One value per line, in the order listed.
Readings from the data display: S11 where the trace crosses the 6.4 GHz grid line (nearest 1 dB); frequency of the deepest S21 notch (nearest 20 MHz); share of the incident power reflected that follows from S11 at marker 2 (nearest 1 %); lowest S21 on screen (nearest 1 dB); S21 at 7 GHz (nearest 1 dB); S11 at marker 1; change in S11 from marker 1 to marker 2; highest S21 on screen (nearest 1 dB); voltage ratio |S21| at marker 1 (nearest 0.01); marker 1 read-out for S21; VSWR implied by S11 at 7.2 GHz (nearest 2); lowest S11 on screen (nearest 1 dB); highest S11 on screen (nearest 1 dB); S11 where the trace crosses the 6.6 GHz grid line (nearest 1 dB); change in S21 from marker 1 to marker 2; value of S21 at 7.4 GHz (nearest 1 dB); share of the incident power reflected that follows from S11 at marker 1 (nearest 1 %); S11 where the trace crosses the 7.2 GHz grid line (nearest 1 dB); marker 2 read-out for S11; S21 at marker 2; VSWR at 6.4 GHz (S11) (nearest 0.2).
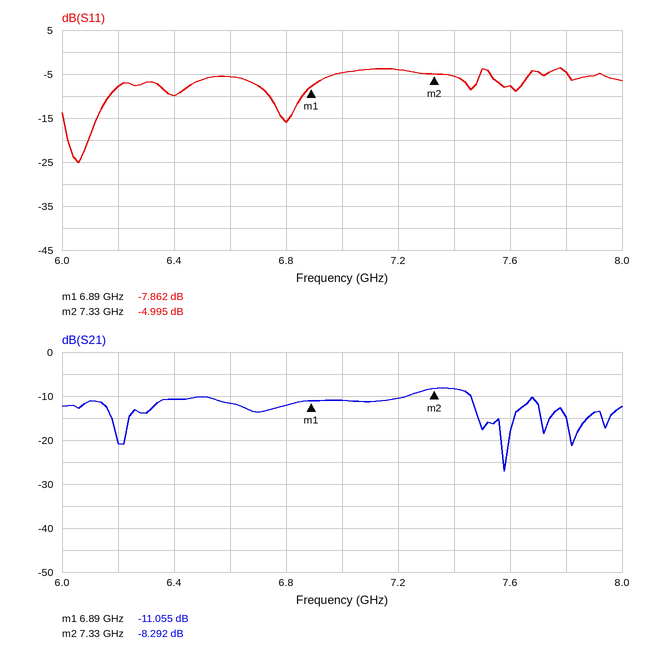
-10 dB
7.58 GHz
32 %
-27 dB
-11 dB
-7.862 dB
2.867 dB
-8 dB
0.28
-11.055 dB
4
-25 dB
-4 dB
-6 dB
2.763 dB
-8 dB
16 %
-4 dB
-4.995 dB
-8.292 dB
2.0
